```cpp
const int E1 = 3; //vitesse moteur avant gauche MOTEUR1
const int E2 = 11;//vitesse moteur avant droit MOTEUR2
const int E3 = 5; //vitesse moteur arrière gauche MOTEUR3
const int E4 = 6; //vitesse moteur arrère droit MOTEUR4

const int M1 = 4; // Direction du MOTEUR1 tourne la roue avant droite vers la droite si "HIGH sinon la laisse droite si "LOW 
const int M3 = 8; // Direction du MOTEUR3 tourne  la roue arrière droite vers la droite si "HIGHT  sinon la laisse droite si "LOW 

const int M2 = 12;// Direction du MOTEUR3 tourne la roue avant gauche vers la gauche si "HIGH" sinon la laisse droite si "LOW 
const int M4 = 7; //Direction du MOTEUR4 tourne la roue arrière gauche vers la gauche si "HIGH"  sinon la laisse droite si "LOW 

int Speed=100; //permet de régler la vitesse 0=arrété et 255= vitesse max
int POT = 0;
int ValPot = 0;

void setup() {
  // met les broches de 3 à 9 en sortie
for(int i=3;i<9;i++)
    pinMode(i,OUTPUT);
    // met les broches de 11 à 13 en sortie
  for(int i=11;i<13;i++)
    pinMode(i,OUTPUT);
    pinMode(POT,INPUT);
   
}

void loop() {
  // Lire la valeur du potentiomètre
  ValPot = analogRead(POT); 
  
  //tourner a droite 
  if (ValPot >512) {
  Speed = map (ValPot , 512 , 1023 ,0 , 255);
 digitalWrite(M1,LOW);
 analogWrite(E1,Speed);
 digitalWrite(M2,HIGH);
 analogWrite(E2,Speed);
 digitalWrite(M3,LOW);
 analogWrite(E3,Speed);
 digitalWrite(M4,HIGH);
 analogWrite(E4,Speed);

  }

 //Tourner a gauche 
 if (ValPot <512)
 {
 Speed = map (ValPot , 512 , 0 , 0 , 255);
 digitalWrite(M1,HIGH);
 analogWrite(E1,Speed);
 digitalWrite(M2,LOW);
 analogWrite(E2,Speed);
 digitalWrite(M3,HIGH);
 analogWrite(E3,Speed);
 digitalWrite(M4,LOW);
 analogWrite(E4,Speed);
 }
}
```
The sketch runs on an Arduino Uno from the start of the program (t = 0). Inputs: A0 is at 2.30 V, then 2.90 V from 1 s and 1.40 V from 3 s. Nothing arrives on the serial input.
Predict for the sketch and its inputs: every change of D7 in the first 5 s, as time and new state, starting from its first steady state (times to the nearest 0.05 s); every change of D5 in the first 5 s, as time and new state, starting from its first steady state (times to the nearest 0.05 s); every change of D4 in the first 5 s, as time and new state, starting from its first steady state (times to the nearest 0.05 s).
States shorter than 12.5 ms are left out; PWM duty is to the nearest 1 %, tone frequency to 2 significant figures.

0 s low; 1 s high; 3 s low
0 s PWM 8 %; 1 s PWM 16 %; 3 s PWM 44 %
0 s high; 1 s low; 3 s high
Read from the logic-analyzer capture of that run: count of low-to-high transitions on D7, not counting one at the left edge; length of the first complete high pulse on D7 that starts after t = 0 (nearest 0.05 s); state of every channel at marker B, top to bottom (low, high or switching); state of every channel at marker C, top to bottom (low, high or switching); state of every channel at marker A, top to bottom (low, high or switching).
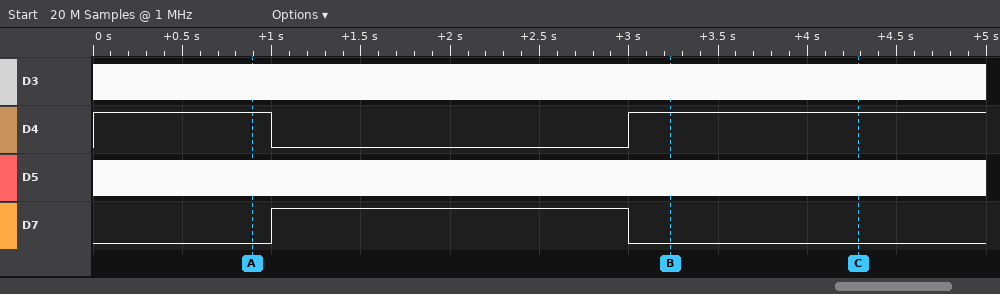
1
2.00 s
D3 switching, D4 high, D5 switching, D7 low
D3 switching, D4 high, D5 switching, D7 low
D3 switching, D4 high, D5 switching, D7 low
